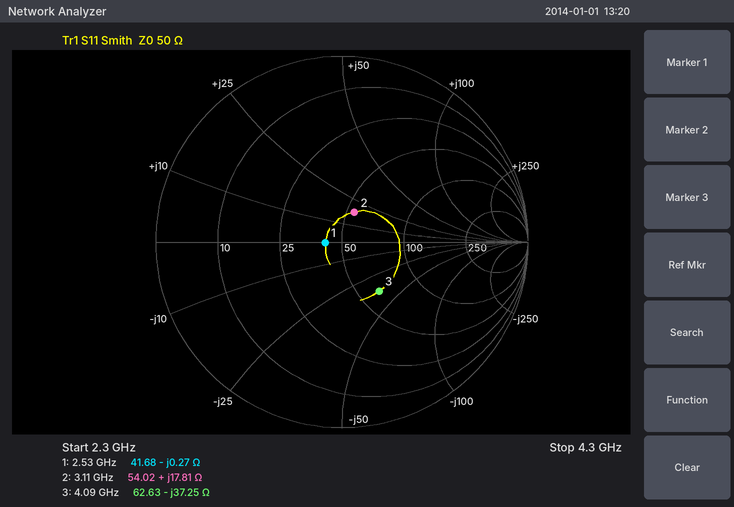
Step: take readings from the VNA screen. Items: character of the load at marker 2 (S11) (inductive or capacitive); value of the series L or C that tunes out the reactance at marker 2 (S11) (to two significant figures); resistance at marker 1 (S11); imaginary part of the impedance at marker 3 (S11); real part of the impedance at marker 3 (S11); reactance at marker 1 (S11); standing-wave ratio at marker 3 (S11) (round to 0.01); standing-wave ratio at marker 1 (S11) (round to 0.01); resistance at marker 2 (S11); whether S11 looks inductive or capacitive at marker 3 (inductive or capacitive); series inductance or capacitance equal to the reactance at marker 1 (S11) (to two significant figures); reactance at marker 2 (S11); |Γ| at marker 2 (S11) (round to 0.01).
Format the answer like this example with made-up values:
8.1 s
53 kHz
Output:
inductive
2.9 pF
41.68 Ω
-37.25 Ω
62.63 Ω
-0.27 Ω
1.99
1.20
54.02 Ω
capacitive
230 pF
+17.81 Ω
0.17
